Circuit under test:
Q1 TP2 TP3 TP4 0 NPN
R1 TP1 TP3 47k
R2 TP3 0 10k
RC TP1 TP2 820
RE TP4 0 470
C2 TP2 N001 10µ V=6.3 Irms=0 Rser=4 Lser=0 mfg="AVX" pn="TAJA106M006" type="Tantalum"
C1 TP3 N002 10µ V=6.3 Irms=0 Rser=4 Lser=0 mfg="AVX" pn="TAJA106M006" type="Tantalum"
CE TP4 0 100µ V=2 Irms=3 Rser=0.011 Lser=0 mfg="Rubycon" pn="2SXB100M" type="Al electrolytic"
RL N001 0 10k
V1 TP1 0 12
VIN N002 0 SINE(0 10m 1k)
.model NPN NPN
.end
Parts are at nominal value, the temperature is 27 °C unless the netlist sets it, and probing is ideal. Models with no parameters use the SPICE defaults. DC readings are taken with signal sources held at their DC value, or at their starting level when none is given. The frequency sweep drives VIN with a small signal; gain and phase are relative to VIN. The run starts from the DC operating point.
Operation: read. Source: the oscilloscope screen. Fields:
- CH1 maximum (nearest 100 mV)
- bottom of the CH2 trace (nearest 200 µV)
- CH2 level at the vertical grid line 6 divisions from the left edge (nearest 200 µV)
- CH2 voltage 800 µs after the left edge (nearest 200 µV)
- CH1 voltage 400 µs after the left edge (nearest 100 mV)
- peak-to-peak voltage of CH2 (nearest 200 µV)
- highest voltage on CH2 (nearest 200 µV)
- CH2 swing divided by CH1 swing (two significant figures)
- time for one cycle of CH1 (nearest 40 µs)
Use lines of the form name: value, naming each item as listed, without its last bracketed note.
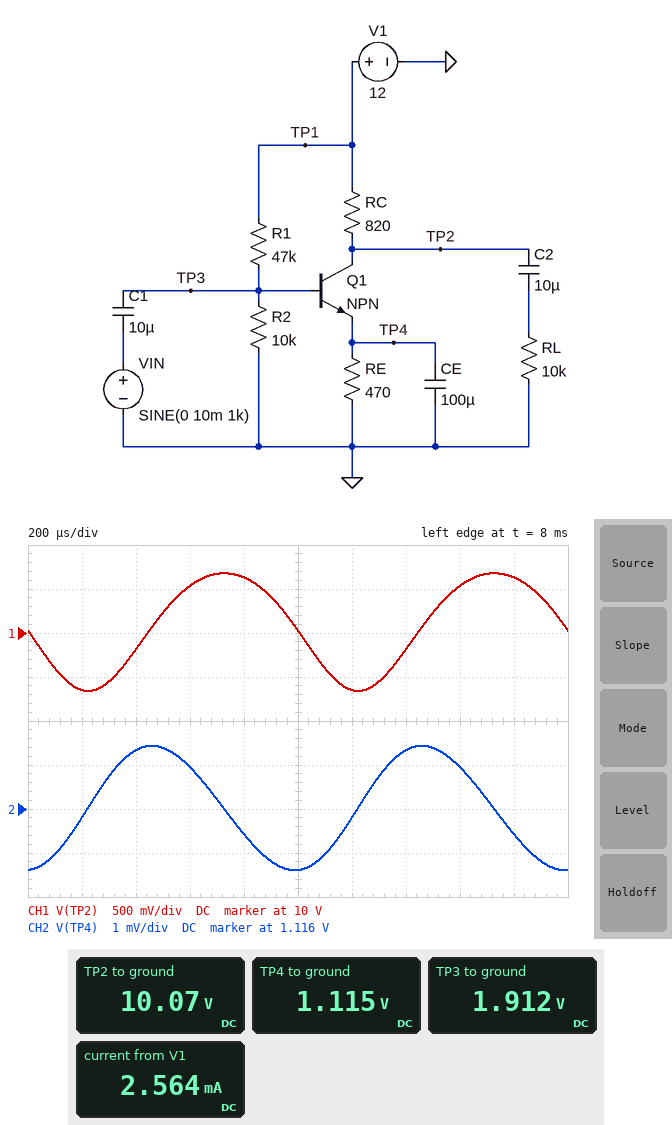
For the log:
CH1 maximum: 10.7 V
bottom of the CH2 trace: 1.1146 V
CH2 level at the vertical grid line 6 divisions from the left edge: 1.1158 V
CH2 voltage 800 µs after the left edge: 1.1154 V
CH1 voltage 400 µs after the left edge: 9.8 V
peak-to-peak voltage of CH2: 2.8 mV
highest voltage on CH2: 1.1174 V
CH2 swing divided by CH1 swing: 0.0021
time for one cycle of CH1: 1.00 ms
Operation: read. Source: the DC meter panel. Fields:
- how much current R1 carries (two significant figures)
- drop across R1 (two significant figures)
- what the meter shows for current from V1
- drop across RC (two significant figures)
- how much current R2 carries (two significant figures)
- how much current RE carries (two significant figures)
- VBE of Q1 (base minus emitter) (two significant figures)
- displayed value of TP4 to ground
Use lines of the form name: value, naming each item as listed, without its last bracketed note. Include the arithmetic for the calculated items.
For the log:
how much current R1 carries: (12 V - 1.912 V) / 47 kΩ = 210 µA
drop across R1: 12 V - 1.912 V = 10 V
what the meter shows for current from V1: 2.564 mA
drop across RC: 12 V - 10.07 V = 1.9 V
how much current R2 carries: (1.912 V) / 10 kΩ = 190 µA
how much current RE carries: (1.115 V) / 470 Ω = 2.4 mA
VBE of Q1 (base minus emitter): 1.912 V - 1.115 V = 800 mV
displayed value of TP4 to ground: 1.115 V
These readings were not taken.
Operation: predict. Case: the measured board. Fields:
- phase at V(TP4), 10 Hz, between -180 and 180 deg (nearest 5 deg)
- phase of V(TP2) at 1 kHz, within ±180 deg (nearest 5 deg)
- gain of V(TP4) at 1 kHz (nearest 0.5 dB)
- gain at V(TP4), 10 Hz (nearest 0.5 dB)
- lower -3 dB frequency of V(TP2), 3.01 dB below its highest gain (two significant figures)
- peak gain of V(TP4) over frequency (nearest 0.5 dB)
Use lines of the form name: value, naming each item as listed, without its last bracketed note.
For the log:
phase at V(TP4), 10 Hz, between -180 and 180 deg: 10 deg
phase of V(TP2) at 1 kHz, within ±180 deg: -170 deg
gain of V(TP4) at 1 kHz: -17.0 dB
gain at V(TP4), 10 Hz: -1.0 dB
lower -3 dB frequency of V(TP2), 3.01 dB below its highest gain: 160 Hz
peak gain of V(TP4) over frequency: -1.0 dB
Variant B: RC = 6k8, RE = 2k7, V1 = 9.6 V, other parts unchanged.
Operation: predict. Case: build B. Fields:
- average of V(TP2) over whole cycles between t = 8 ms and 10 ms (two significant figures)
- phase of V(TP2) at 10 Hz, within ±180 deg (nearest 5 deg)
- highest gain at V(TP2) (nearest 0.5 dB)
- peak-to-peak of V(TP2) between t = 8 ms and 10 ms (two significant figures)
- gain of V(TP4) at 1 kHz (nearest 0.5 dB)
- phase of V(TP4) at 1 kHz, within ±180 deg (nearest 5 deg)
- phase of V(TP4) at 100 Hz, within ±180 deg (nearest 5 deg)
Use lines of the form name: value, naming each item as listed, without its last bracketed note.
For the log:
average of V(TP2) over whole cycles between t = 8 ms and 10 ms: 7.3 V
phase of V(TP2) at 10 Hz, within ±180 deg: -110 deg
highest gain at V(TP2): 34.5 dB
peak-to-peak of V(TP2) between t = 8 ms and 10 ms: 1.0 V
gain of V(TP4) at 1 kHz: -33.5 dB
phase of V(TP4) at 1 kHz, within ±180 deg: -90 deg
phase of V(TP4) at 100 Hz, within ±180 deg: -75 deg
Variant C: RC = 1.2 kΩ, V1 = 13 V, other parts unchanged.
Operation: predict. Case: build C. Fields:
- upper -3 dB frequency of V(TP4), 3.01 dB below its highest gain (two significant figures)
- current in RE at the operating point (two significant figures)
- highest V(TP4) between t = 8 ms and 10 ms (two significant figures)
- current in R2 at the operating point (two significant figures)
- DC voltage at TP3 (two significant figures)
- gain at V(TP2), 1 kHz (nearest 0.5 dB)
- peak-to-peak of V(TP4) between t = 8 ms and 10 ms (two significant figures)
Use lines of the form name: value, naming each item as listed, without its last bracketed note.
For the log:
upper -3 dB frequency of V(TP4), 3.01 dB below its highest gain: 190 Hz
current in RE at the operating point: 2.7 mA
highest V(TP4) between t = 8 ms and 10 ms: 1.3 V
current in R2 at the operating point: 210 µA
DC voltage at TP3: 2.1 V
gain at V(TP2), 1 kHz: 40.5 dB
peak-to-peak of V(TP4) between t = 8 ms and 10 ms: 3.2 mV
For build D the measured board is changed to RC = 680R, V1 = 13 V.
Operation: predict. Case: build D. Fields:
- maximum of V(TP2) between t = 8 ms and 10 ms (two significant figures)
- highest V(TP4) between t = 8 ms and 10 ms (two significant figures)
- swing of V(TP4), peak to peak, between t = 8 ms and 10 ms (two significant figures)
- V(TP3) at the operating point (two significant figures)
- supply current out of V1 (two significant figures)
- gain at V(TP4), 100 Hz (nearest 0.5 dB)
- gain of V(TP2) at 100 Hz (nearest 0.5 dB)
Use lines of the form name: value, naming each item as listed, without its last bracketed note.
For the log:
maximum of V(TP2) between t = 8 ms and 10 ms: 12 V
highest V(TP4) between t = 8 ms and 10 ms: 1.3 V
swing of V(TP4), peak to peak, between t = 8 ms and 10 ms: 3.2 mV
V(TP3) at the operating point: 2.1 V
supply current out of V1: 2.9 mA
gain at V(TP4), 100 Hz: -2.0 dB
gain of V(TP2) at 100 Hz: 30.0 dB
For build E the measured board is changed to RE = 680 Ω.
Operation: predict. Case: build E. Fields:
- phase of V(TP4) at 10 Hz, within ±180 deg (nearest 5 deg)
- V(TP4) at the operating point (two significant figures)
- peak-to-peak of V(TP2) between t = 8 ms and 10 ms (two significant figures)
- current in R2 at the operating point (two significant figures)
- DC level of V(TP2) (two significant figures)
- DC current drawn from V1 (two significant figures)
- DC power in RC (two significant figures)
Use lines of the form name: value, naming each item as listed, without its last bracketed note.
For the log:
phase of V(TP4) at 10 Hz, within ±180 deg: 5 deg
V(TP4) at the operating point: 1.2 V
peak-to-peak of V(TP2) between t = 8 ms and 10 ms: 980 mV
current in R2 at the operating point: 200 µA
DC level of V(TP2): 11 V
DC current drawn from V1: 1.9 mA
DC power in RC: 2.4 mW
